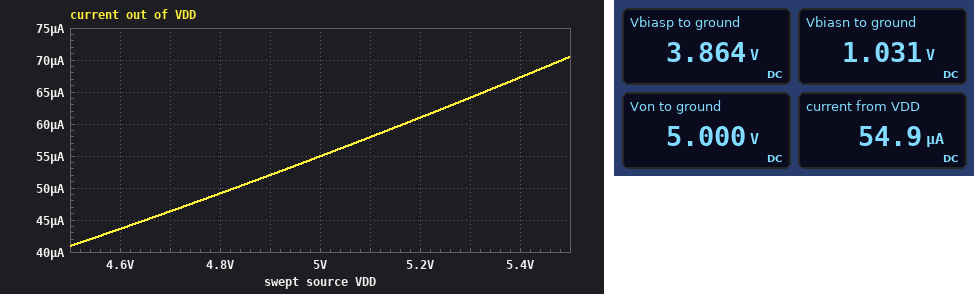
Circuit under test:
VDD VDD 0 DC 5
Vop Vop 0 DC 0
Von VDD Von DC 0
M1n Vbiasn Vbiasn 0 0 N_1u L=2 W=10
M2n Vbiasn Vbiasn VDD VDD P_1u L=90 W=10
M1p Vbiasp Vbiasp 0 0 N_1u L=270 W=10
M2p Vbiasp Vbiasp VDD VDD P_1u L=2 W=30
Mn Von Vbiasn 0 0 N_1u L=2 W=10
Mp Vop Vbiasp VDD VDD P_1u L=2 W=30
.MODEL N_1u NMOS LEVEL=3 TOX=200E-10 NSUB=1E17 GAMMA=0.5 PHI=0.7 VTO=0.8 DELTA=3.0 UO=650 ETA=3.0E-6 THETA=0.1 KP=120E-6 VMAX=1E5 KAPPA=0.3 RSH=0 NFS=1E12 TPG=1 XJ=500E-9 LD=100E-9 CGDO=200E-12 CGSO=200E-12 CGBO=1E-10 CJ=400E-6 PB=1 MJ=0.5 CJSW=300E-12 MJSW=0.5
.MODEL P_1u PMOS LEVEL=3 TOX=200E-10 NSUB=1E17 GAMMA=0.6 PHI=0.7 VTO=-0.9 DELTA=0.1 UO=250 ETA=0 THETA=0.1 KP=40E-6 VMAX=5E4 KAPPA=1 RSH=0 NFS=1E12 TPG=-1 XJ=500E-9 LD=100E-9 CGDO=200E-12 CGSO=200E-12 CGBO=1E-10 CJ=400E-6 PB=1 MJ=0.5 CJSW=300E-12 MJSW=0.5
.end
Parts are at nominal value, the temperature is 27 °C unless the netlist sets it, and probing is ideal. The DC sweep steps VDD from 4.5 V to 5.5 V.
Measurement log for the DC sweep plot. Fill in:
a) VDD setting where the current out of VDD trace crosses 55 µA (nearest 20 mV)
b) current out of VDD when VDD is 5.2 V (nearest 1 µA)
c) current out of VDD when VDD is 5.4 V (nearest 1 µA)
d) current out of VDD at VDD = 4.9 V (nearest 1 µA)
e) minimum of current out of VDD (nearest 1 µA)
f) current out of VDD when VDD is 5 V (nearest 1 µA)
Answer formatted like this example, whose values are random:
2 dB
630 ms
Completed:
5.00 V
61 µA
67 µA
52 µA
41 µA
55 µA
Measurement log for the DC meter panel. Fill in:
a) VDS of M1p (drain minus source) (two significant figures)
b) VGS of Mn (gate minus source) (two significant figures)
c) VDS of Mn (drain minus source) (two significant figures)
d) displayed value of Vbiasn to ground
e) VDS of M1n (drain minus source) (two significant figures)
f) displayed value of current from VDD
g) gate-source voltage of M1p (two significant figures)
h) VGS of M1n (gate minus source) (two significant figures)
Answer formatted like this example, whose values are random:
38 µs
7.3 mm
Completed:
3.9 V
1.0 V
5.0 V
1.031 V
1.0 V
54.9 µA
3.9 V
1.0 V
